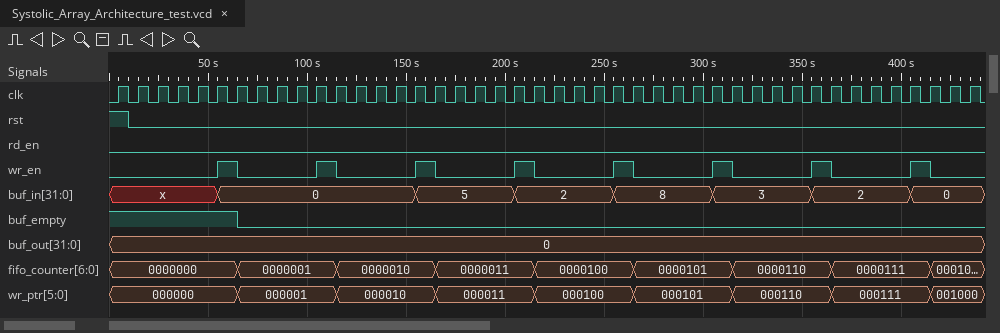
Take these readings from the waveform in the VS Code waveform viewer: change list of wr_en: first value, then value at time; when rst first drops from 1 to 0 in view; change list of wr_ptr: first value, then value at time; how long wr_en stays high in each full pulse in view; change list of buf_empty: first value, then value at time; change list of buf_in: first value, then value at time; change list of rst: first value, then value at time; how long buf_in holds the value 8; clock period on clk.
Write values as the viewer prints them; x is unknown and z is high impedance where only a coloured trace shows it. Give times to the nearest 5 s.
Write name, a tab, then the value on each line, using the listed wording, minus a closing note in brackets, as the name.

change list of wr_en: first value, then value at time	0, 1 at 55 s, 0 at 65 s, 1 at 105 s, 0 at 115 s, 1 at 155 s, 0 at 165 s, 1 at 205 s, 0 at 215 s, 1 at 255 s, 0 at 265 s, 1 at 305 s, 0 at 315 s, 1 at 355 s, 0 at 365 s, 1 at 405 s, 0 at 415 s
when rst first drops from 1 to 0 in view	10 s
change list of wr_ptr: first value, then value at time	000000, 000001 at 65 s, 000010 at 115 s, 000011 at 165 s, 000100 at 215 s, 000101 at 265 s, 000110 at 315 s, 000111 at 365 s, 001000 at 415 s
how long wr_en stays high in each full pulse in view	10 s, 10 s, 10 s, 10 s, 10 s, 10 s, 10 s, 10 s
change list of buf_empty: first value, then value at time	1, 0 at 65 s
change list of buf_in: first value, then value at time	x, 0 at 55 s, 5 at 155 s, 2 at 205 s, 8 at 255 s, 3 at 305 s, 2 at 355 s, 0 at 405 s
change list of rst: first value, then value at time	1, 0 at 10 s
how long buf_in holds the value 8	50 s
clock period on clk	10 s
